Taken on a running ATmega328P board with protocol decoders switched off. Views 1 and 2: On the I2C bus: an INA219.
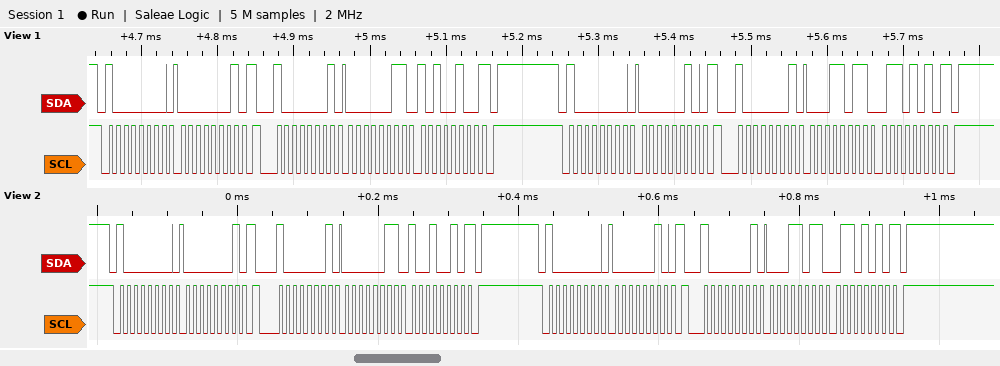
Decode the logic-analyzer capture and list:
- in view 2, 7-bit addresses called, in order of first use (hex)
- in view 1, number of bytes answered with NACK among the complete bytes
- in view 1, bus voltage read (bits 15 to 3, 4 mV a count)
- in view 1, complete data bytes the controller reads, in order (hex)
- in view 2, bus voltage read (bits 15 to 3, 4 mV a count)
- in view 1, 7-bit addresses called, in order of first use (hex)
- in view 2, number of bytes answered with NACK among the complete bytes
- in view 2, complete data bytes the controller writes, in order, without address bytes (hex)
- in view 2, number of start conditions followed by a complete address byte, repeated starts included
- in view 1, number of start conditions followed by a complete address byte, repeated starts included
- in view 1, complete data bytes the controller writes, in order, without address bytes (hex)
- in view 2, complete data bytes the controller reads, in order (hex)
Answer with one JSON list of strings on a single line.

["0x40", "2", "3.508 V", "03 A4 1B 6A", "3.508 V", "0x40", "2", "01 02", "4", "4", "01 02", "03 92 1B 6A"]
